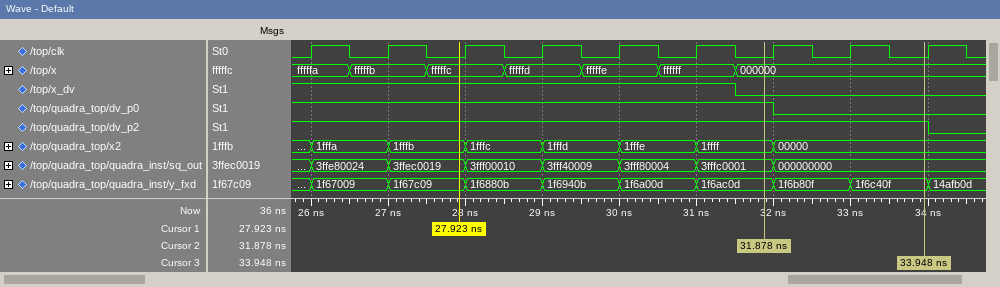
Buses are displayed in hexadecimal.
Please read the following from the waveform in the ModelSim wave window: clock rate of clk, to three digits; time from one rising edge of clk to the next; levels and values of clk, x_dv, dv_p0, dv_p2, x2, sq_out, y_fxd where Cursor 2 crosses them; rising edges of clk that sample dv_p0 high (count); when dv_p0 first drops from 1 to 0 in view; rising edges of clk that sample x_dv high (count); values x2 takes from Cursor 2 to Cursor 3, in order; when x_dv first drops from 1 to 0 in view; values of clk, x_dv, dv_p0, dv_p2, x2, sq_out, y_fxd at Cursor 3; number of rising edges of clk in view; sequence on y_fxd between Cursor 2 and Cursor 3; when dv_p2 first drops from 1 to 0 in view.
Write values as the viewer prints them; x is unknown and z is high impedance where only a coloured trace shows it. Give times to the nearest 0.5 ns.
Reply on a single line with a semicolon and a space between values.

1.00 GHz; 1 ns; clk=0, x_dv=0, dv_p0=1, dv_p2=1, x2=1ffff, sq_out=3fffc0001, y_fxd=1f6ac0d; 7; 32 ns; 6; 1ffff, 00000; 31.5 ns; clk=0, x_dv=0, dv_p0=0, dv_p2=1, x2=00000, sq_out=000000000, y_fxd=1f6c40f; 9; 1f6ac0d, 1f6b80f, 1f6c40f; 34 ns
